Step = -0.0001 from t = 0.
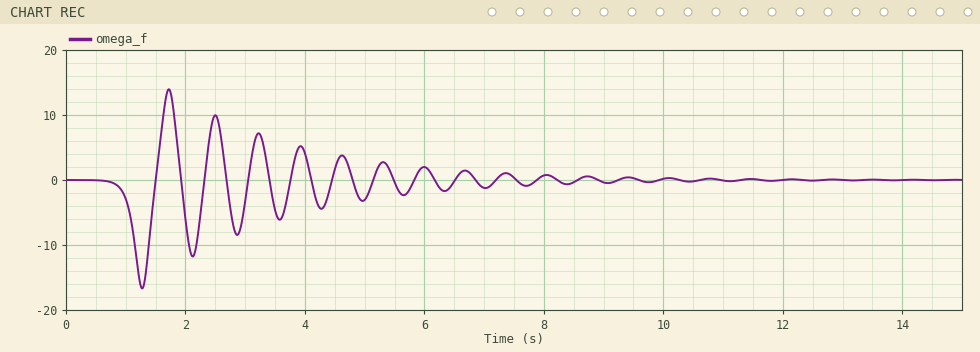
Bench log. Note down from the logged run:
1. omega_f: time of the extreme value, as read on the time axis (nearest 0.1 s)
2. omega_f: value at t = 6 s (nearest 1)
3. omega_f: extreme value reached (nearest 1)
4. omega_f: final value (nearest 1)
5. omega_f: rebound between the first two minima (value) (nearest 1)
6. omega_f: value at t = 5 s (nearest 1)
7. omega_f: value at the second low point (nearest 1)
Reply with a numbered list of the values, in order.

1. 1.3 s
2. 2
3. -17
4. 0
5. 14
6. -3
7. -12
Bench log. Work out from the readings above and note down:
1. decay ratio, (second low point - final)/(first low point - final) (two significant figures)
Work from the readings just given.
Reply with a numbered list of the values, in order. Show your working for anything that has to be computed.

1. (-12 - 0) / (-17 - 0) = 0.71
